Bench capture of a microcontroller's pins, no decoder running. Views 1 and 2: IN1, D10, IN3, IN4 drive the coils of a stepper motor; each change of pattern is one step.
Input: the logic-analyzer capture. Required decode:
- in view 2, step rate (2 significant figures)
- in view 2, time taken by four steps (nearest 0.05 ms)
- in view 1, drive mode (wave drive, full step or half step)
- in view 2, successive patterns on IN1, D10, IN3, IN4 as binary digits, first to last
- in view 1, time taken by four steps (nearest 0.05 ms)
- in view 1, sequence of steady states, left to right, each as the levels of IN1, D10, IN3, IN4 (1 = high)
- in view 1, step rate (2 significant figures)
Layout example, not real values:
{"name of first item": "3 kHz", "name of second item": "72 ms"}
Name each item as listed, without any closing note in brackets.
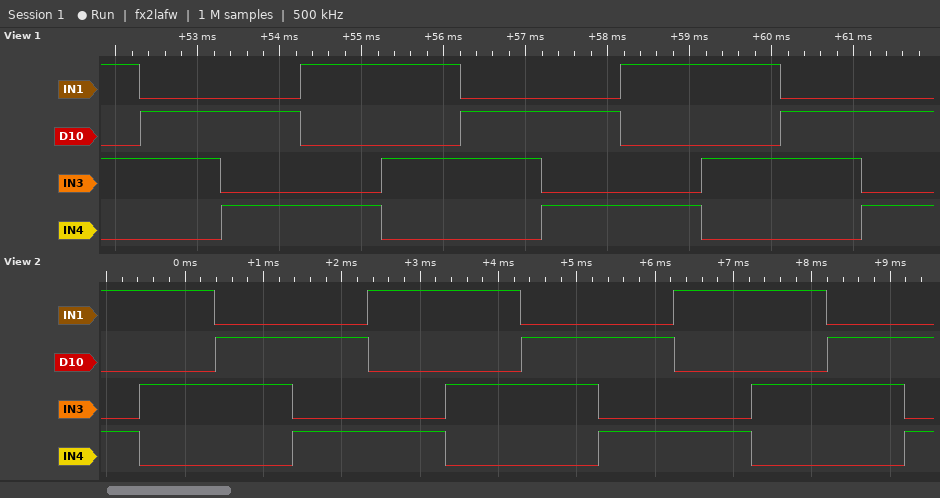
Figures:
{"in view 2, step rate": "1000 steps/s", "in view 2, time taken by four steps": "3.90 ms", "in view 1, drive mode": "full step", "in view 2, successive patterns on IN1, D10, IN3, IN4 as binary digits, first to last": "1001 1010 0110 0101 1001 1010 0110 0101 1001 1010 0110 0101", "in view 1, time taken by four steps": "3.90 ms", "in view 1, sequence of steady states, left to right, each as the levels of IN1, D10, IN3, IN4": "1010 0110 0101 1001 1010 0110 0101 1001 1010 0110 0101", "in view 1, step rate": "1000 steps/s"}
